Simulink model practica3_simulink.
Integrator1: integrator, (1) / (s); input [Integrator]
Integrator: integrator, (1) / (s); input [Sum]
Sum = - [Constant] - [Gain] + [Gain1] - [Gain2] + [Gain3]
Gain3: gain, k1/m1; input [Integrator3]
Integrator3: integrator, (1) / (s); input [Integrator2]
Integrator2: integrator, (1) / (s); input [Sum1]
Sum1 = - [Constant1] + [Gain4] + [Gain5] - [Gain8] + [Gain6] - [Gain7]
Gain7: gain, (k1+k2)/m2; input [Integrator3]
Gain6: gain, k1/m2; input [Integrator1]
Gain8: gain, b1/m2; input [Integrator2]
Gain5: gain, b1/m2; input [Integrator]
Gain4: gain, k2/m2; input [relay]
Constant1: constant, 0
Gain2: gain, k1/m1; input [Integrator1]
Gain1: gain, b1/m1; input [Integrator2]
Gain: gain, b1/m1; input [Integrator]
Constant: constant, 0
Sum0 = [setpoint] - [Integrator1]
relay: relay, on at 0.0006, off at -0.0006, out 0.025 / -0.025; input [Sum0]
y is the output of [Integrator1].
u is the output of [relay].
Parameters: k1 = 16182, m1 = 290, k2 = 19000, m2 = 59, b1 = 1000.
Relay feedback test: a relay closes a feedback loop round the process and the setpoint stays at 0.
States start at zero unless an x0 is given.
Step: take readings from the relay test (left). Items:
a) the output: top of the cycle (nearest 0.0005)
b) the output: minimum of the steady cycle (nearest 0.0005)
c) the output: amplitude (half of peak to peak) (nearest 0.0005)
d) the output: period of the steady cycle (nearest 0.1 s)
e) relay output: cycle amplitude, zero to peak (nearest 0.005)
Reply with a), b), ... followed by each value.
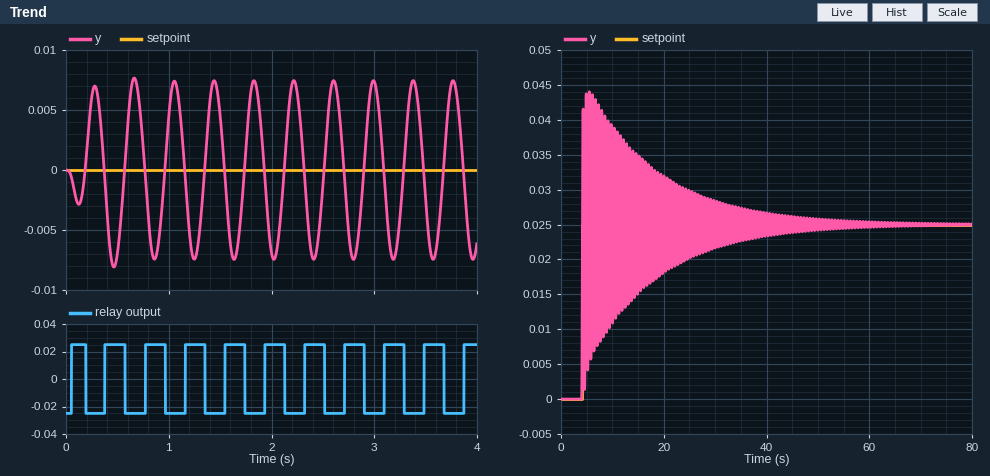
a) 0.0075
b) -0.0075
c) 0.0075
d) 0.4 s
e) 0.025
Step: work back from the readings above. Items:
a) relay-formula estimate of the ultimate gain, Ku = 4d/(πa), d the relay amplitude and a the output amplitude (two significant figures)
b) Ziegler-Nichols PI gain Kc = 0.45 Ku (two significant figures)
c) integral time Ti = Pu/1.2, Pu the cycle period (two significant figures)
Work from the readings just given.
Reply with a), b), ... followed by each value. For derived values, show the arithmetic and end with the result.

a) 4 × 0.025 / (π × 0.0075) = 4.2
b) 0.45 × 4.2 = 1.9
c) 0.4 / 1.2 = 0.33 s
